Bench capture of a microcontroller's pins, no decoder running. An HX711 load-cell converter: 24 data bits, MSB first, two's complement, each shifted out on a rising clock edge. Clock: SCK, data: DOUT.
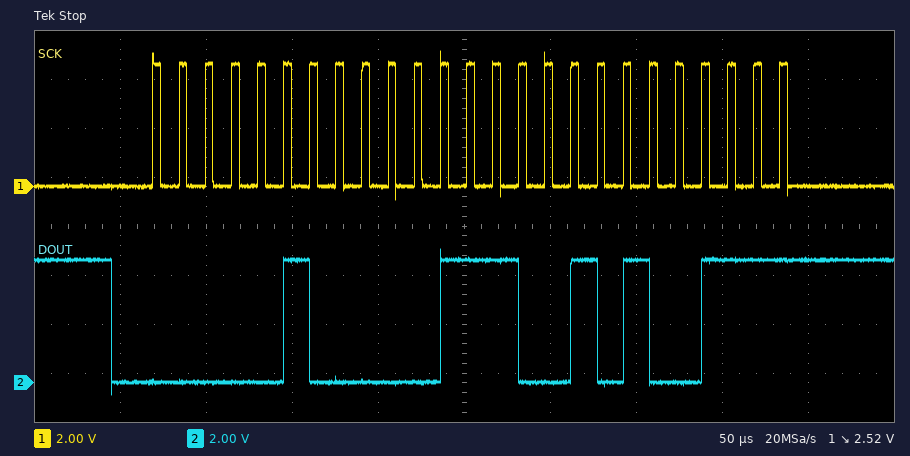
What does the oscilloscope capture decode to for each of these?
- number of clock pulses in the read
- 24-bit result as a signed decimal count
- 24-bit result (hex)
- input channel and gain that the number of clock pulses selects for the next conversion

25
269479
0x041CA7
channel A, gain 128
